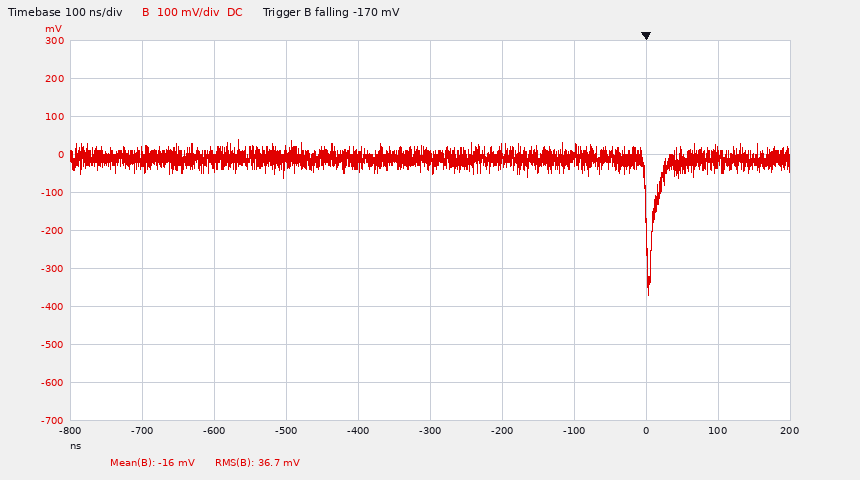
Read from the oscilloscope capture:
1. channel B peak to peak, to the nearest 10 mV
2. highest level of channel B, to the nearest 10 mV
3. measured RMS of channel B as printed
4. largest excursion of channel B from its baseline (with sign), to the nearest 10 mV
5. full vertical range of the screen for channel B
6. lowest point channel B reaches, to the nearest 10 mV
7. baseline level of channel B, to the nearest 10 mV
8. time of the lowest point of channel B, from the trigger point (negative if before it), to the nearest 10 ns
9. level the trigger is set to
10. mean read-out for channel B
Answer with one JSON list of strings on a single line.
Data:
["410 mV", "40 mV", "36.7 mV", "-360 mV", "1 V", "-370 mV", "-10 mV", "0 ns", "-170 mV", "-16 mV"]
